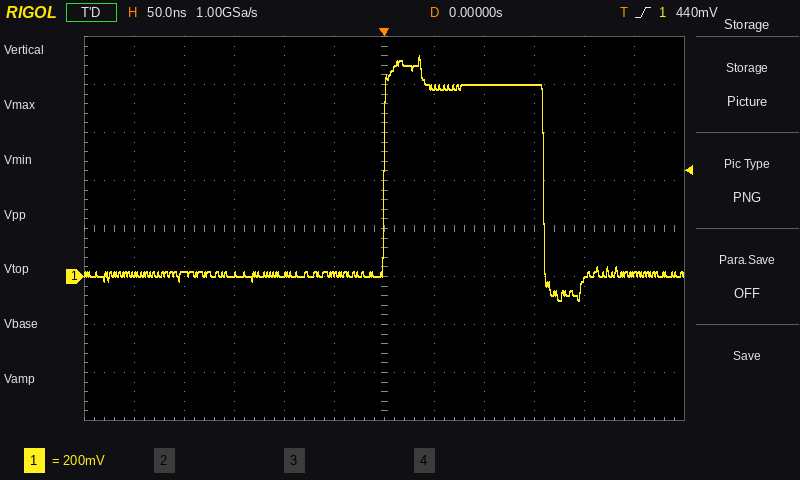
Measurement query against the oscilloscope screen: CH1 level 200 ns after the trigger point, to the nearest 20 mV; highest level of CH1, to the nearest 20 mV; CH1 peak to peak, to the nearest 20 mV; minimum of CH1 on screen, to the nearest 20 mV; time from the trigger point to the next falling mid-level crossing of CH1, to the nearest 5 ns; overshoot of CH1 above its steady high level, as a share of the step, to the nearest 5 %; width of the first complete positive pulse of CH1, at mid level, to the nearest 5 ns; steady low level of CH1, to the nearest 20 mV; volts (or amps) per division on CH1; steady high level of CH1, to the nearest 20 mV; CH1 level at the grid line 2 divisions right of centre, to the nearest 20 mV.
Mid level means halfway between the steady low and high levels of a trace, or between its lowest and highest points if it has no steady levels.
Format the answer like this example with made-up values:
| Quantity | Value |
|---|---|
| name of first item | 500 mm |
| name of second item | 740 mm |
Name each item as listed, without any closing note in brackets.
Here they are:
| Quantity | Value |
|---|---|
| CH1 level 200 ns after the trigger point, to the nearest 20 mV | -20 mV |
| highest level of CH1, to the nearest 20 mV | 920 mV |
| CH1 peak to peak, to the nearest 20 mV | 1.02 V |
| minimum of CH1 on screen, to the nearest 20 mV | -100 mV |
| time from the trigger point to the next falling mid-level crossing of CH1, to the nearest 5 ns | 160 ns |
| overshoot of CH1 above its steady high level, as a share of the step, to the nearest 5 % | 15 % |
| width of the first complete positive pulse of CH1, at mid level, to the nearest 5 ns | 160 ns |
| steady low level of CH1, to the nearest 20 mV | 0 mV |
| volts (or amps) per division on CH1 | 200 mV |
| steady high level of CH1, to the nearest 20 mV | 800 mV |
| CH1 level at the grid line 2 divisions right of centre, to the nearest 20 mV | 800 mV |
